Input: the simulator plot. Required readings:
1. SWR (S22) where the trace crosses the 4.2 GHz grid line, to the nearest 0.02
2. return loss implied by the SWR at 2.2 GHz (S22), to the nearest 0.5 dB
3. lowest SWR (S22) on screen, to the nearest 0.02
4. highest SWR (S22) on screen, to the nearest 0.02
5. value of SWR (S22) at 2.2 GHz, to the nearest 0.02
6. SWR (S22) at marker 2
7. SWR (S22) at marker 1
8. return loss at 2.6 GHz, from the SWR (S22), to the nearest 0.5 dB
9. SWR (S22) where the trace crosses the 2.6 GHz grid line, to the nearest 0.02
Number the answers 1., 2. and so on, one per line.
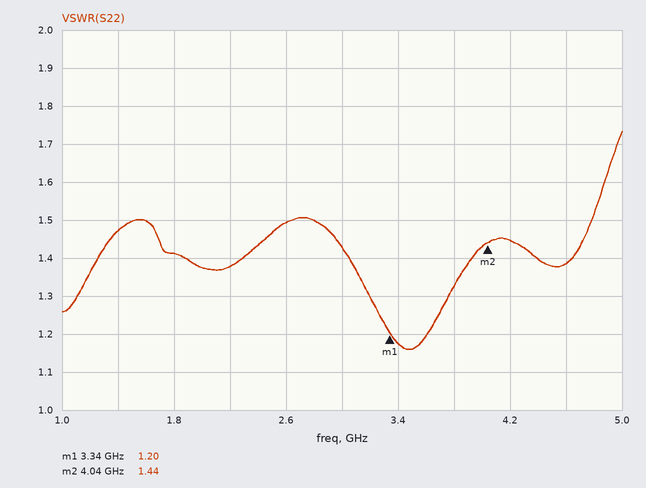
1. 1.44
2. 16.0 dB
3. 1.16
4. 1.74
5. 1.38
6. 1.44
7. 1.20
8. 14.0 dB
9. 1.50
